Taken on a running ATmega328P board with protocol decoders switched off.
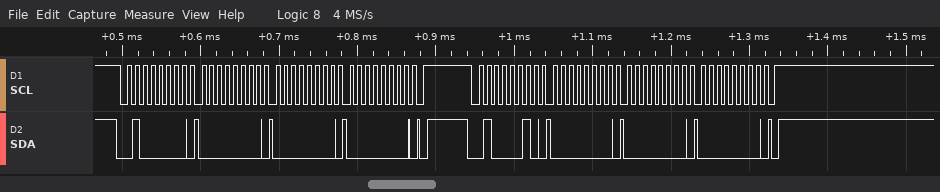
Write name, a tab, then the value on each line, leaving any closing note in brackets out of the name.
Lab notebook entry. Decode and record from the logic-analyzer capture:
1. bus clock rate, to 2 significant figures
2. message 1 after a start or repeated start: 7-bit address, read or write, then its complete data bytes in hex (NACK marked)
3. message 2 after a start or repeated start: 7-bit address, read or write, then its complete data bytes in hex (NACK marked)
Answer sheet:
bus clock rate, to 2 significant figures	100 kHz
message 1 after a start or repeated start: 7-bit address, read or write, then its complete data bytes in hex	0x20 write: 00 00 00
message 2 after a start or repeated start: 7-bit address, read or write, then its complete data bytes in hex	0x21 write: 00 00 00
